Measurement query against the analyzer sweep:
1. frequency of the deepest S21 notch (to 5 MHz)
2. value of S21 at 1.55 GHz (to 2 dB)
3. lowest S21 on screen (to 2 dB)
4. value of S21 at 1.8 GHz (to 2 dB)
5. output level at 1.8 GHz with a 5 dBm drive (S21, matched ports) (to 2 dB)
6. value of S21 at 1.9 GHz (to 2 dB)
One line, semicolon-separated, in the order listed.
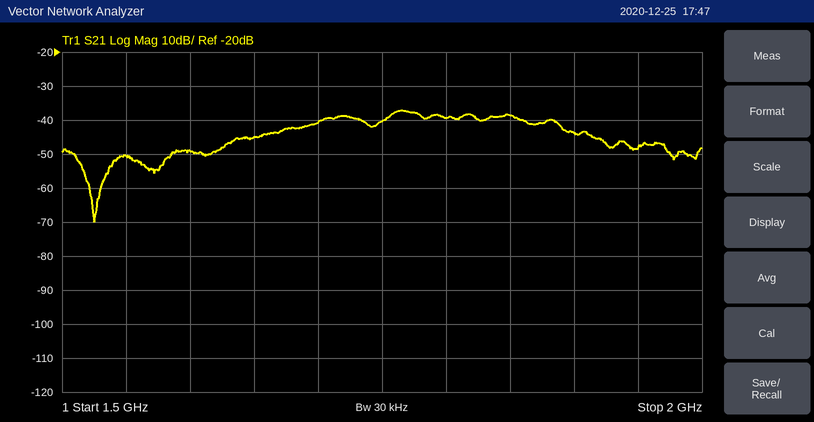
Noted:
1.525 GHz; -50 dB; -70 dB; -40 dB; -34 dBm; -44 dB
